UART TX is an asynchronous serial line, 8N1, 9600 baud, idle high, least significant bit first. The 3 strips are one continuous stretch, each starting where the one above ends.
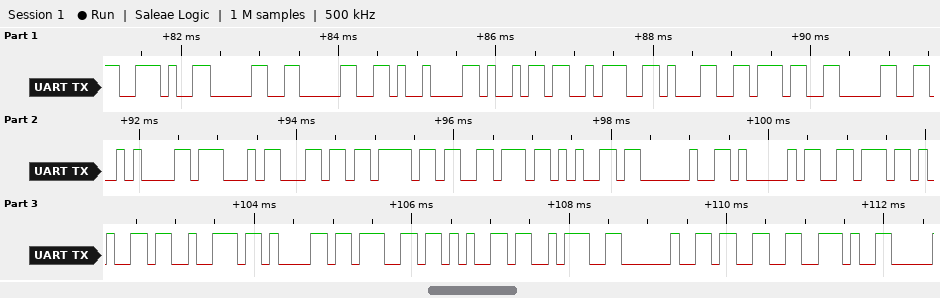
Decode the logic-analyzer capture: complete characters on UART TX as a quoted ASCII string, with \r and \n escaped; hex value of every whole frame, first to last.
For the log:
".00\ti:170\nGlove Average: 3."
2E 30 30 09 69 3A 31 37 30 0A 47 6C 6F 76 65 20 41 76 65 72 61 67 65 3A 20 33 2E
